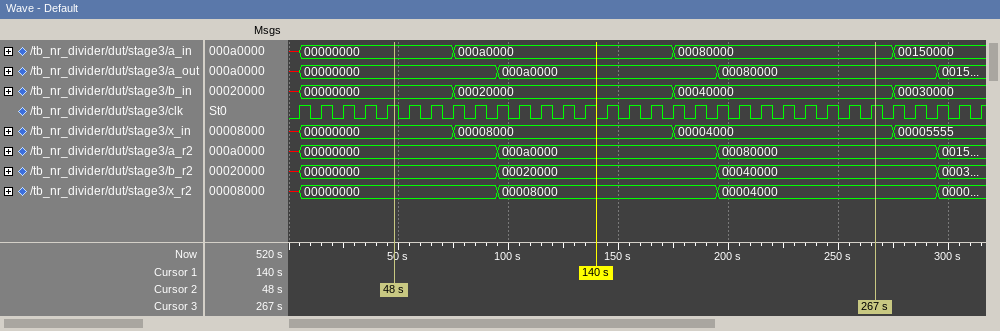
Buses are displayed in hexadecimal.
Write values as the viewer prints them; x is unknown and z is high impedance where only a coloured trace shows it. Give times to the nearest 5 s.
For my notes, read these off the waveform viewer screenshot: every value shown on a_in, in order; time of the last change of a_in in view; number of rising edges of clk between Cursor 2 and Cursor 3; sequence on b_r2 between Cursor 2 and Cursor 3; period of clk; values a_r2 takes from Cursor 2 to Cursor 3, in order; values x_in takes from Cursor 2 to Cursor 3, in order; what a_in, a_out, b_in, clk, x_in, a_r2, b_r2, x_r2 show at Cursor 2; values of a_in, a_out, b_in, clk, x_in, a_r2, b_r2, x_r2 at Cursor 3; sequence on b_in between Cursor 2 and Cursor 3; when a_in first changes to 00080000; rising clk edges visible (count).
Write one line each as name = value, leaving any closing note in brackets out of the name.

every value shown on a_in, in order = x, 00000000, 000a0000, 00080000, 00150000
time of the last change of a_in in view = 275 s
number of rising edges of clk between Cursor 2 and Cursor 3 = 22
sequence on b_r2 between Cursor 2 and Cursor 3 = 00000000, 00020000, 00040000
period of clk = 10 s
values a_r2 takes from Cursor 2 to Cursor 3, in order = 00000000, 000a0000, 00080000
values x_in takes from Cursor 2 to Cursor 3, in order = 00000000, 00008000, 00004000
what a_in, a_out, b_in, clk, x_in, a_r2, b_r2, x_r2 show at Cursor 2 = a_in=00000000, a_out=00000000, b_in=00000000, clk=1, x_in=00000000, a_r2=00000000, b_r2=00000000, x_r2=00000000
values of a_in, a_out, b_in, clk, x_in, a_r2, b_r2, x_r2 at Cursor 3 = a_in=00080000, a_out=00080000, b_in=00040000, clk=1, x_in=00004000, a_r2=00080000, b_r2=00040000, x_r2=00004000
sequence on b_in between Cursor 2 and Cursor 3 = 00000000, 00020000, 00040000
when a_in first changes to 00080000 = 175 s
rising clk edges visible = 32
